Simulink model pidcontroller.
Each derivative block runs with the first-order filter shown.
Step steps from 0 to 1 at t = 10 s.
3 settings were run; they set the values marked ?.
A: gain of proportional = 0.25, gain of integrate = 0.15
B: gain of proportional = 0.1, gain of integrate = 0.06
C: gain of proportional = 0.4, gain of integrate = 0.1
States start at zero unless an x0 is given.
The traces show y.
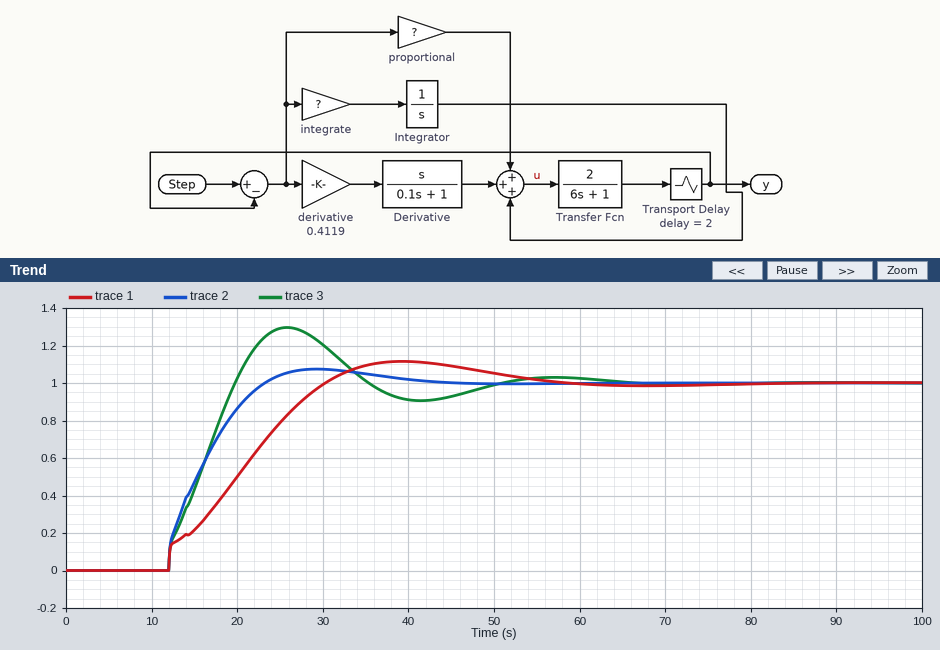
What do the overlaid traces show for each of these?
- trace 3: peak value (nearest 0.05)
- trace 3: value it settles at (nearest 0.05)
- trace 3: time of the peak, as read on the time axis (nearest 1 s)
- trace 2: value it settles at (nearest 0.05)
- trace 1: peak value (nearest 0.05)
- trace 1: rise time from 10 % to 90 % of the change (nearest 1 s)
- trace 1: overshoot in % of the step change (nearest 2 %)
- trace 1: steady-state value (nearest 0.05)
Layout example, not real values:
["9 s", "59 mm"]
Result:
["1.30", "1.00", "26 s", "1.00", "1.10", "15 s", "12 %", "1.00"]
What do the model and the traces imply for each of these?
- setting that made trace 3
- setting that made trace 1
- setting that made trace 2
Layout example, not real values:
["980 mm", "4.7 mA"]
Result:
["A", "B", "C"]
